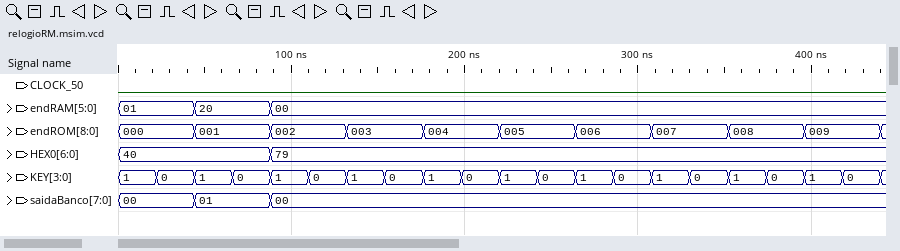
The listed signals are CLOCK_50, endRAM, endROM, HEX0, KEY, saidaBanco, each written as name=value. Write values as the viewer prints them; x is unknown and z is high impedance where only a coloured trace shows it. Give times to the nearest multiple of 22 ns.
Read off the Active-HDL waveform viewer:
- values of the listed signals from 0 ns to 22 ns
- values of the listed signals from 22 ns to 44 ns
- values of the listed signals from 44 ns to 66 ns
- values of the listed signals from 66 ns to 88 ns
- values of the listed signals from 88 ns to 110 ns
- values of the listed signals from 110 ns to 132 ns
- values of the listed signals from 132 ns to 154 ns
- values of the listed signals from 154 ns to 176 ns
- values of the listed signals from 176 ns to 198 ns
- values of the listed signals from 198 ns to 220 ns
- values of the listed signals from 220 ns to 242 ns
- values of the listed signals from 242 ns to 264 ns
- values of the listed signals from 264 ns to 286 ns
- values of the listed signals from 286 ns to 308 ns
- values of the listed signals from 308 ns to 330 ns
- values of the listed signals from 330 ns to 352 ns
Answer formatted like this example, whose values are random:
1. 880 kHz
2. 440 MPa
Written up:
1. CLOCK_50=0, endRAM=01, endROM=000, HEX0=40, KEY=1, saidaBanco=00
2. CLOCK_50=0, endRAM=01, endROM=000, HEX0=40, KEY=0, saidaBanco=00
3. CLOCK_50=0, endRAM=20, endROM=001, HEX0=40, KEY=1, saidaBanco=01
4. CLOCK_50=0, endRAM=20, endROM=001, HEX0=40, KEY=0, saidaBanco=01
5. CLOCK_50=0, endRAM=00, endROM=002, HEX0=79, KEY=1, saidaBanco=00
6. CLOCK_50=0, endRAM=00, endROM=002, HEX0=79, KEY=0, saidaBanco=00
7. CLOCK_50=0, endRAM=00, endROM=003, HEX0=79, KEY=1, saidaBanco=00
8. CLOCK_50=0, endRAM=00, endROM=003, HEX0=79, KEY=0, saidaBanco=00
9. CLOCK_50=0, endRAM=00, endROM=004, HEX0=79, KEY=1, saidaBanco=00
10. CLOCK_50=0, endRAM=00, endROM=004, HEX0=79, KEY=0, saidaBanco=00
11. CLOCK_50=0, endRAM=00, endROM=005, HEX0=79, KEY=1, saidaBanco=00
12. CLOCK_50=0, endRAM=00, endROM=005, HEX0=79, KEY=0, saidaBanco=00
13. CLOCK_50=0, endRAM=00, endROM=006, HEX0=79, KEY=1, saidaBanco=00
14. CLOCK_50=0, endRAM=00, endROM=006, HEX0=79, KEY=0, saidaBanco=00
15. CLOCK_50=0, endRAM=00, endROM=007, HEX0=79, KEY=1, saidaBanco=00
16. CLOCK_50=0, endRAM=00, endROM=007, HEX0=79, KEY=0, saidaBanco=00
